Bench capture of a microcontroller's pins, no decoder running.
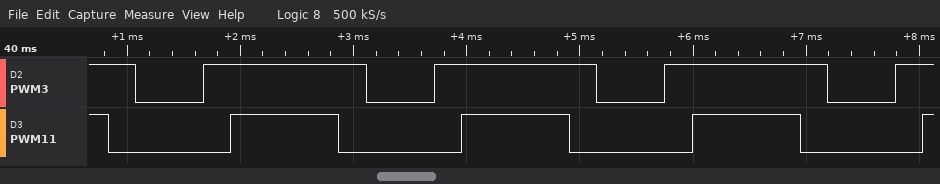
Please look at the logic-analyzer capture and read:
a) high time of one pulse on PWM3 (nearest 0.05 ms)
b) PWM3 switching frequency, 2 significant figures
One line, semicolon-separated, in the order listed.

1.45 ms; 490 Hz
